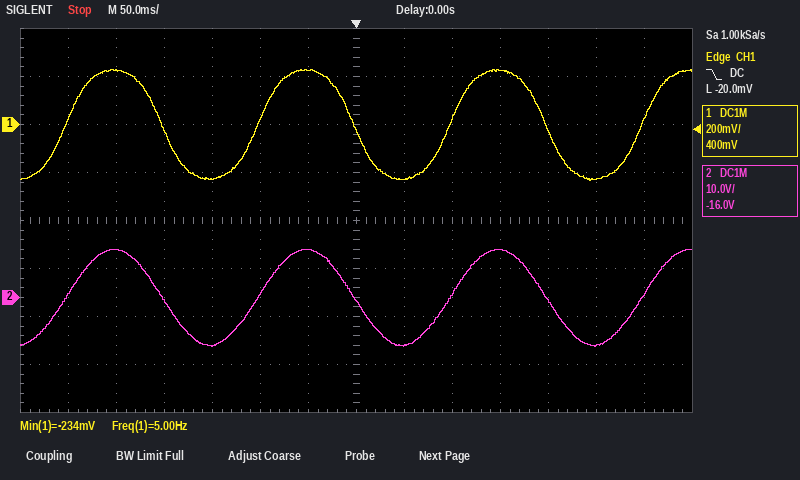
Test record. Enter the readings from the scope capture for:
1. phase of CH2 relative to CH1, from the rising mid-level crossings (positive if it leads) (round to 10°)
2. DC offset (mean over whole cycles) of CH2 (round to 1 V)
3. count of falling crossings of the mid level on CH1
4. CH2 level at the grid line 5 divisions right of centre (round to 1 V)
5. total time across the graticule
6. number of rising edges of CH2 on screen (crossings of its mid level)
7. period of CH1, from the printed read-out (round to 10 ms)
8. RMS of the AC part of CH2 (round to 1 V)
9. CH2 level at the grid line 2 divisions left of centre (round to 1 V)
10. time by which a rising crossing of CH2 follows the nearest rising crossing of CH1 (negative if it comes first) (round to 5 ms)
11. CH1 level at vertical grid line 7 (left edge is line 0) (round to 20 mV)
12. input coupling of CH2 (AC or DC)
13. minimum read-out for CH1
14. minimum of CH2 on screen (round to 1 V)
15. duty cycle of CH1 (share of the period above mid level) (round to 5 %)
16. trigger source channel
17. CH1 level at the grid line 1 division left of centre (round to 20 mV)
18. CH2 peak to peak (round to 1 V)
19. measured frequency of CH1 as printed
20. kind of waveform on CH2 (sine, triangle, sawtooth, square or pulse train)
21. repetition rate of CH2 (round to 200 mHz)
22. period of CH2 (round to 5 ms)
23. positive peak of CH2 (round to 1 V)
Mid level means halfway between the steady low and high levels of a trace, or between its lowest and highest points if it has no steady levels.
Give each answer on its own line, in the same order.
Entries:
0°
0 V
3
-10 V
700 ms
4
200 ms
7 V
1 V
0 ms
-20 mV
DC
-234 mV
-10 V
50 %
CH1
220 mV
20 V
5.00 Hz
sine
5.0 Hz
200 ms
10 V
